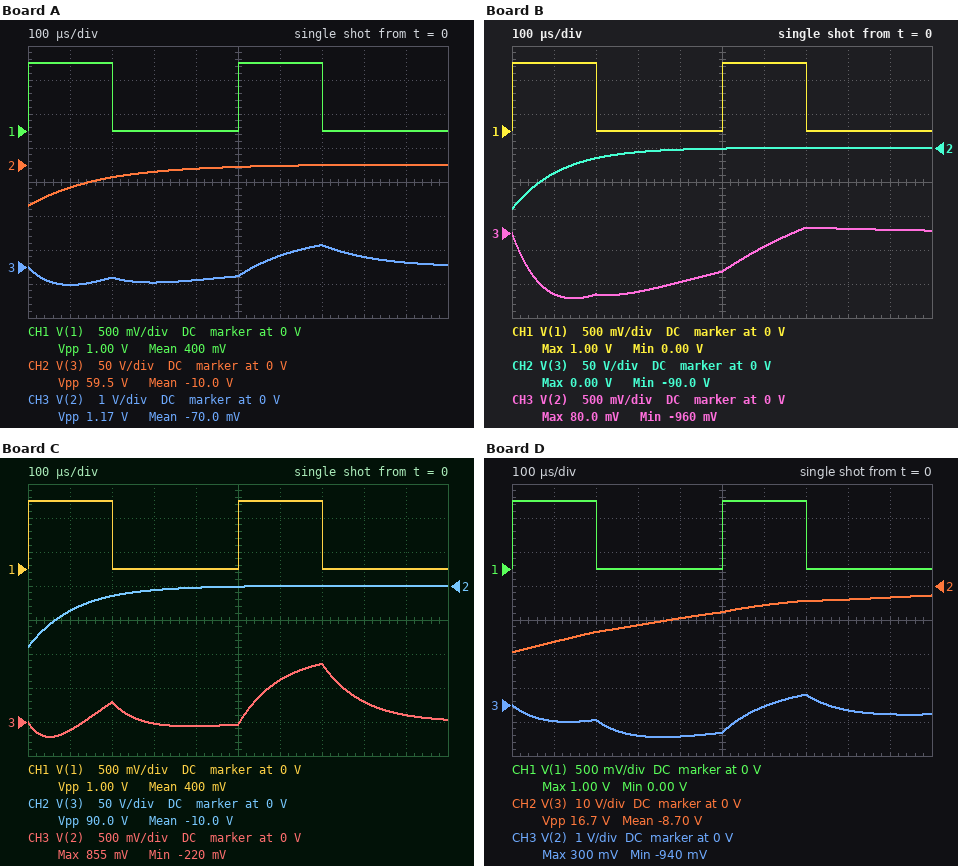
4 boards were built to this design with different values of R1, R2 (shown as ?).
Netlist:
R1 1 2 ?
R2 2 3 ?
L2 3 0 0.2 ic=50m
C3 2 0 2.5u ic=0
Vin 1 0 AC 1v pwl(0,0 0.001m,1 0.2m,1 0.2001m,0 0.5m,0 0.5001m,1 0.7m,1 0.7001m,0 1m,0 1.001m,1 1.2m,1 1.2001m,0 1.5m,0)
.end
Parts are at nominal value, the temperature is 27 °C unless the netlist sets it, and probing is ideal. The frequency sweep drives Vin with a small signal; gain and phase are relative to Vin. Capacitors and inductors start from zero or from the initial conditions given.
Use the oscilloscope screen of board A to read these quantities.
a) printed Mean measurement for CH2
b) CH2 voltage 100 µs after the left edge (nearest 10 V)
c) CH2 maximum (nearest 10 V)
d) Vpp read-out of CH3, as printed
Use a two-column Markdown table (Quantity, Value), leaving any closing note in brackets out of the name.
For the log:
| Quantity | Value |
|---|---|
| printed Mean measurement for CH2 | -10.0 V |
| CH2 voltage 100 µs after the left edge | -30 V |
| CH2 maximum | 0 V |
| Vpp read-out of CH3, as printed | 1.17 V |
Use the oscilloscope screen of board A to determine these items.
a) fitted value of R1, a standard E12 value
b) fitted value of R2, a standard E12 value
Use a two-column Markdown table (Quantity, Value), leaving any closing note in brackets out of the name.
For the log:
| Quantity | Value |
|---|---|
| fitted value of R1, a standard E12 value | 56 Ω |
| fitted value of R2, a standard E12 value | 1.2 kΩ |
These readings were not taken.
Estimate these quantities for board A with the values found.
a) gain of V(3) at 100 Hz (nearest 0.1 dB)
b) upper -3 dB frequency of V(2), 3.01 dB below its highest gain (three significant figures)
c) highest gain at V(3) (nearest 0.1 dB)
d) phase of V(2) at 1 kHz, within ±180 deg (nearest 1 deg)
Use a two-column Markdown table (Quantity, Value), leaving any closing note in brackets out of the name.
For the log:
| Quantity | Value |
|---|---|
| gain of V(3) at 100 Hz | -20.1 dB |
| upper -3 dB frequency of V(2), 3.01 dB below its highest gain | 1.25 kHz |
| highest gain at V(3) | -5.3 dB |
| phase of V(2) at 1 kHz, within ±180 deg | -40 deg |
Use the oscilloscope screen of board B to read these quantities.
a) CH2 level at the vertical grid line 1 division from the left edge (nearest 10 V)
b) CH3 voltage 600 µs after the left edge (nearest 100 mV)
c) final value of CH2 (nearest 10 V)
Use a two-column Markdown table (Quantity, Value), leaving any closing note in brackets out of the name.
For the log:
| Quantity | Value |
|---|---|
| CH2 level at the vertical grid line 1 division from the left edge | -40 V |
| CH3 voltage 600 µs after the left edge | -200 mV |
| final value of CH2 | 0 V |
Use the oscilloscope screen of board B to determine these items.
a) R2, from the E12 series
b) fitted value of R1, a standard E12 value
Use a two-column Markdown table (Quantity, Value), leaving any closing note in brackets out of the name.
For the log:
| Quantity | Value |
|---|---|
| R2, from the E12 series | 1.8 kΩ |
| fitted value of R1, a standard E12 value | 150 Ω |
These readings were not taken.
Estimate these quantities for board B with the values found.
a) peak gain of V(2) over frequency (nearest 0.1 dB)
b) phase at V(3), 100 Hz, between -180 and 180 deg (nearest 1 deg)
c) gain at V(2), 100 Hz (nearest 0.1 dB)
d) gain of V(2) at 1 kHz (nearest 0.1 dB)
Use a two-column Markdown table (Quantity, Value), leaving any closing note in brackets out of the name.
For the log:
| Quantity | Value |
|---|---|
| peak gain of V(2) over frequency | -0.7 dB |
| phase at V(3), 100 Hz, between -180 and 180 deg | 74 deg |
| gain at V(2), 100 Hz | -0.9 dB |
| gain of V(2) at 1 kHz | -8.1 dB |
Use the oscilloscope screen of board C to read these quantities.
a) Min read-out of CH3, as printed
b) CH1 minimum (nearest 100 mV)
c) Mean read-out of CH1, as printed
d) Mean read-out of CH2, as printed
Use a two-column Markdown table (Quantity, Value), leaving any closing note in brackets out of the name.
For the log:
| Quantity | Value |
|---|---|
| Min read-out of CH3, as printed | -220 mV |
| CH1 minimum | 0 V |
| Mean read-out of CH1, as printed | 400 mV |
| Mean read-out of CH2, as printed | -10.0 V |
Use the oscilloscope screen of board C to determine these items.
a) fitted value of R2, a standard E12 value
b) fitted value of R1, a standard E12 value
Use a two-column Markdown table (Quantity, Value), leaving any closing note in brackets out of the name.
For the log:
| Quantity | Value |
|---|---|
| fitted value of R2, a standard E12 value | 1.8 kΩ |
| fitted value of R1, a standard E12 value | 39 Ω |
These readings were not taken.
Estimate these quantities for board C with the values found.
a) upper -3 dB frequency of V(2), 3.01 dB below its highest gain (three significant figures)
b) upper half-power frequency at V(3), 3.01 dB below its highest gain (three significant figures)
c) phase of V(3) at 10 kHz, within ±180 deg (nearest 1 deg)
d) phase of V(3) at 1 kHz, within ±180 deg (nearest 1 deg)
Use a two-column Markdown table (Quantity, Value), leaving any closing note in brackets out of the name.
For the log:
| Quantity | Value |
|---|---|
| upper -3 dB frequency of V(2), 3.01 dB below its highest gain | 1.71 kHz |
| upper half-power frequency at V(3), 3.01 dB below its highest gain | 3.71 kHz |
| phase of V(3) at 10 kHz, within ±180 deg | -73 deg |
| phase of V(3) at 1 kHz, within ±180 deg | 24 deg |
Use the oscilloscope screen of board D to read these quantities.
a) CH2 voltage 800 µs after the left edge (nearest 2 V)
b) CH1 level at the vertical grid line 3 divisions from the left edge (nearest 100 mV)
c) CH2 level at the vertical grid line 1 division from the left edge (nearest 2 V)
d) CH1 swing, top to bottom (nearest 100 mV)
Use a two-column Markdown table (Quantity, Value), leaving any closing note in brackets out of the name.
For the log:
| Quantity | Value |
|---|---|
| CH2 voltage 800 µs after the left edge | -4 V |
| CH1 level at the vertical grid line 3 divisions from the left edge | 0 V |
| CH2 level at the vertical grid line 1 division from the left edge | -16 V |
| CH1 swing, top to bottom | 1.0 V |
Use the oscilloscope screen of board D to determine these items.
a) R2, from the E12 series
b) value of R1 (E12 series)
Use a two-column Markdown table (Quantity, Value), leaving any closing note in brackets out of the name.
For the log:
| Quantity | Value |
|---|---|
| R2, from the E12 series | 390 Ω |
| value of R1 | 39 Ω |
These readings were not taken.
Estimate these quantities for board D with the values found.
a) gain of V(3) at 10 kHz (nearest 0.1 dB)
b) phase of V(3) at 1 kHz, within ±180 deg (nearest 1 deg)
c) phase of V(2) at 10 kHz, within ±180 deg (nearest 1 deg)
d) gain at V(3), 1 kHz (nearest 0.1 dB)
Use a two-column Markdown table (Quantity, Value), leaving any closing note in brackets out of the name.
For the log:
| Quantity | Value |
|---|---|
| gain of V(3) at 10 kHz | -15.9 dB |
| phase of V(3) at 1 kHz, within ±180 deg | -13 deg |
| phase of V(2) at 10 kHz, within ±180 deg | -81 deg |
| gain at V(3), 1 kHz | -1.7 dB |
